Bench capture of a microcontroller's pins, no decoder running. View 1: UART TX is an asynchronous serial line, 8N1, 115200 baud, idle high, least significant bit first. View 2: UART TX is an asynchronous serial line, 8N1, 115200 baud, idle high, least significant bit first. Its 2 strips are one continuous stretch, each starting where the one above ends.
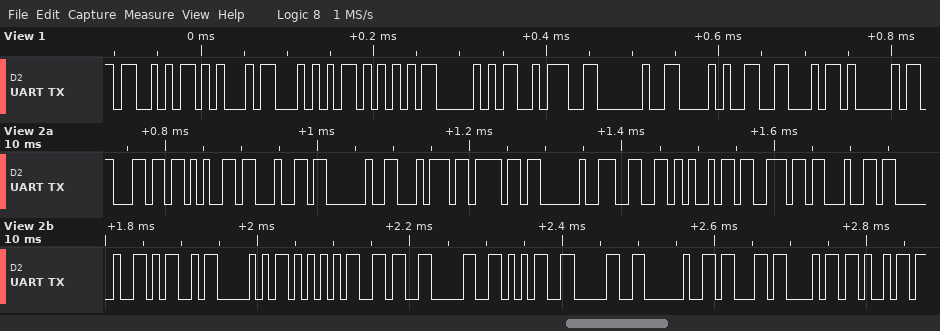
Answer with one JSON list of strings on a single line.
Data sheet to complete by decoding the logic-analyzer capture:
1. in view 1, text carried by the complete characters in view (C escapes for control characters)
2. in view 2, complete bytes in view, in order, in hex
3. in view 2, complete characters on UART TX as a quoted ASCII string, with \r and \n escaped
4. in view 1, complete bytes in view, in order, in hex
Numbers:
["\"SETUP: (FA\"", "6C 65 64 20 74 6F 20 66 69 6E 64 20 4D 50 55 36 30 35 30 20 63 68 69", "\"led to find MPU6050 chi\"", "53 45 54 55 50 3A 20 28 46 41"]
